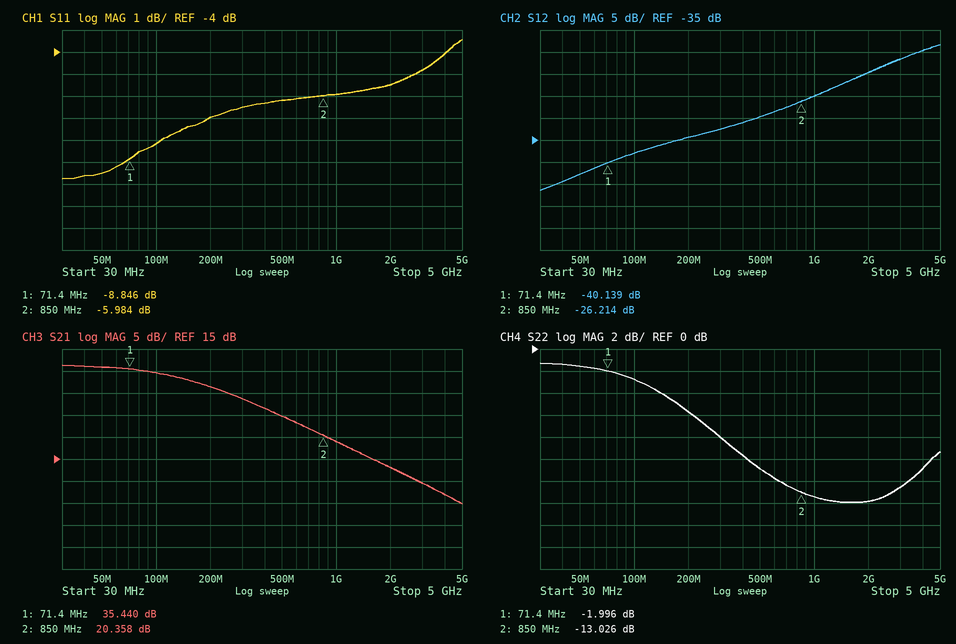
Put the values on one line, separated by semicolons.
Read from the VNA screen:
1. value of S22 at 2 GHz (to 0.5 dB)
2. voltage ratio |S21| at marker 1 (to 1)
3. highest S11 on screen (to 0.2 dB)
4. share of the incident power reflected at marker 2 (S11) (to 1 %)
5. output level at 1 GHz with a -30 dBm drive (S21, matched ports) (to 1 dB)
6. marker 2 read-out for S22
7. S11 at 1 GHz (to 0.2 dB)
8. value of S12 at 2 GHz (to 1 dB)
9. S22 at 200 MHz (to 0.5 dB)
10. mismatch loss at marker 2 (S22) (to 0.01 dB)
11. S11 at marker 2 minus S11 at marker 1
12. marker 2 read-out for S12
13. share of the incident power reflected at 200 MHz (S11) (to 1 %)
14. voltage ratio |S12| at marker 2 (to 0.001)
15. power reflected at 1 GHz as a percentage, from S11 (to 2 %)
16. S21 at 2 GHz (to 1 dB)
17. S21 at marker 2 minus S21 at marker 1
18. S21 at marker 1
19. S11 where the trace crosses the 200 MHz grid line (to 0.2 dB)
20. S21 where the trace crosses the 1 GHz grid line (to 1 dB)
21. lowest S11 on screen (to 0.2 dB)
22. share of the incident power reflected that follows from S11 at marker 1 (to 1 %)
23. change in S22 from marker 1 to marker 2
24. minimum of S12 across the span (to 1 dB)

-14.0 dB; 59; -3.4 dB; 25 %; -11 dBm; -13.026 dB; -6.0 dB; -20 dB; -5.5 dB; 0.22 dB; 2.862 dB; -26.214 dB; 20 %; 0.049; 26 %; 13 dB; -15.082 dB; 35.440 dB; -7.0 dB; 19 dB; -9.8 dB; 13 %; -11.030 dB; -46 dB
